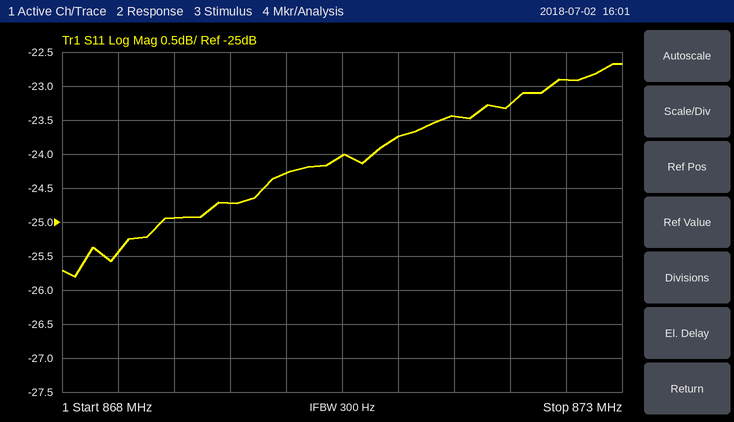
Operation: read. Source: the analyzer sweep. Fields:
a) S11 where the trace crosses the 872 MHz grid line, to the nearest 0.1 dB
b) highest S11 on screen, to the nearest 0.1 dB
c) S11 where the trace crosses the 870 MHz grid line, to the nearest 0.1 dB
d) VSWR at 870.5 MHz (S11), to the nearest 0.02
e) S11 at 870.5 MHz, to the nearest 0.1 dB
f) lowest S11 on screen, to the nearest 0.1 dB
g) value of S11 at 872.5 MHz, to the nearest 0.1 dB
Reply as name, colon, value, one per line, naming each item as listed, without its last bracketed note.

S11 where the trace crosses the 872 MHz grid line, to the nearest 0.1 dB: -23.3 dB
highest S11 on screen, to the nearest 0.1 dB: -22.7 dB
S11 where the trace crosses the 870 MHz grid line, to the nearest 0.1 dB: -24.3 dB
VSWR at 870.5 MHz (S11), to the nearest 0.02: 1.14
S11 at 870.5 MHz, to the nearest 0.1 dB: -24.0 dB
lowest S11 on screen, to the nearest 0.1 dB: -25.8 dB
value of S11 at 872.5 MHz, to the nearest 0.1 dB: -22.9 dB
